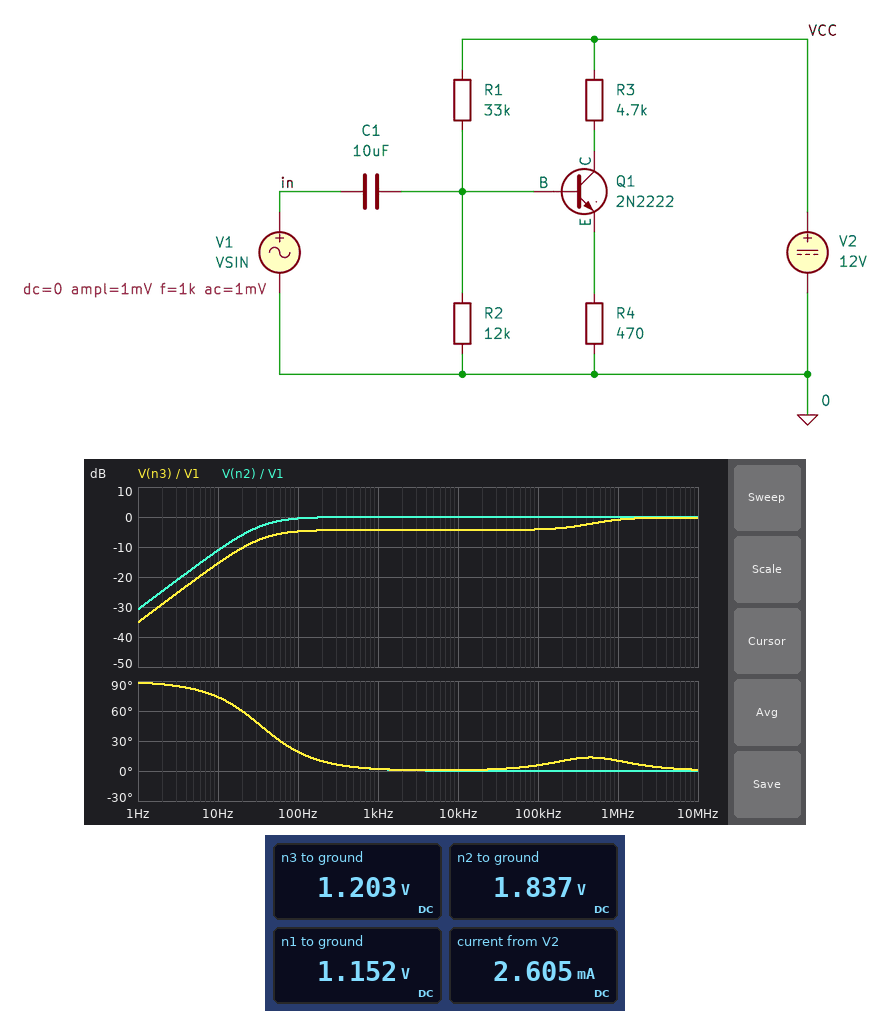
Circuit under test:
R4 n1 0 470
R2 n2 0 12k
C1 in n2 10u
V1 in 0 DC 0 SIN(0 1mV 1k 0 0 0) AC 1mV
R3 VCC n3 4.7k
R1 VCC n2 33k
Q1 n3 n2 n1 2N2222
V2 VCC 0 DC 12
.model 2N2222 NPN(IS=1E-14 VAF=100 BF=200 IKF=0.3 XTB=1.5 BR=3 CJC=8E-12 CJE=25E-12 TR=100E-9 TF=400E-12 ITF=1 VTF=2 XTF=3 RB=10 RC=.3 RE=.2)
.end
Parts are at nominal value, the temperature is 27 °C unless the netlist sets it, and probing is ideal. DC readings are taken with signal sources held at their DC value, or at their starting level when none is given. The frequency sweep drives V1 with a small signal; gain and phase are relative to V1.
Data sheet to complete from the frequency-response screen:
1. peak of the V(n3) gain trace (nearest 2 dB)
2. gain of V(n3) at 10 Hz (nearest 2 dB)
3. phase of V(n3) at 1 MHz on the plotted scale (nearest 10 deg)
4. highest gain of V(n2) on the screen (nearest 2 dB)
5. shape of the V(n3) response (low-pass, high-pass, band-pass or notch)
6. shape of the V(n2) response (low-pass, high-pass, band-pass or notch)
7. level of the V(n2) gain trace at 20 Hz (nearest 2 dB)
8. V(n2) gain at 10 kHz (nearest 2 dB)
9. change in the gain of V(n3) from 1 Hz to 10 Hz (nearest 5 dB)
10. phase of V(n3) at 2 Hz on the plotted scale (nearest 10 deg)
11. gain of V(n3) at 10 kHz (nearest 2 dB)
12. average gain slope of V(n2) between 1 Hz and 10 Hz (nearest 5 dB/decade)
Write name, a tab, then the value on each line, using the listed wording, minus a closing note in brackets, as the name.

peak of the V(n3) gain trace	0 dB
gain of V(n3) at 10 Hz	-16 dB
phase of V(n3) at 1 MHz on the plotted scale	10 deg
highest gain of V(n2) on the screen	0 dB
shape of the V(n3) response	high-pass
shape of the V(n2) response	high-pass
level of the V(n2) gain trace at 20 Hz	-6 dB
V(n2) gain at 10 kHz	0 dB
change in the gain of V(n3) from 1 Hz to 10 Hz	20 dB
phase of V(n3) at 2 Hz on the plotted scale	90 deg
gain of V(n3) at 10 kHz	-4 dB
average gain slope of V(n2) between 1 Hz and 10 Hz	20 dB/decade
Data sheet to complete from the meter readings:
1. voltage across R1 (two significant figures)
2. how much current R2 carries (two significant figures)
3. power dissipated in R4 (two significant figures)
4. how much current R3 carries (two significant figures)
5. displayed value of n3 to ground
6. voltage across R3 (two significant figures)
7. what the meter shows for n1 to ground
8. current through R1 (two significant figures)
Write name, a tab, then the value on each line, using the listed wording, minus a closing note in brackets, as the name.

voltage across R1	10 V
how much current R2 carries	150 µA
power dissipated in R4	2.8 mW
how much current R3 carries	2.3 mA
displayed value of n3 to ground	1.203 V
voltage across R3	11 V
what the meter shows for n1 to ground	1.152 V
current through R1	310 µA
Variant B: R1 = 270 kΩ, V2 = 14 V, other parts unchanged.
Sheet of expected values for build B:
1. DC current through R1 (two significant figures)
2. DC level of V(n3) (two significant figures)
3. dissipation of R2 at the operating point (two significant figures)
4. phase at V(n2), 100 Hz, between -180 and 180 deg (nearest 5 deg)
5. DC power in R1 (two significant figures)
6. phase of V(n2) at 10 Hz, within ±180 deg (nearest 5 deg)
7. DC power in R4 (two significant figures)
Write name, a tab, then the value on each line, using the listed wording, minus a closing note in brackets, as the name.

DC current through R1	50 µA
DC level of V(n3)	14 V
dissipation of R2 at the operating point	29 µW
phase at V(n2), 100 Hz, between -180 and 180 deg	0 deg
DC power in R1	670 µW
phase of V(n2) at 10 Hz, within ±180 deg	10 deg
DC power in R4	980 nW
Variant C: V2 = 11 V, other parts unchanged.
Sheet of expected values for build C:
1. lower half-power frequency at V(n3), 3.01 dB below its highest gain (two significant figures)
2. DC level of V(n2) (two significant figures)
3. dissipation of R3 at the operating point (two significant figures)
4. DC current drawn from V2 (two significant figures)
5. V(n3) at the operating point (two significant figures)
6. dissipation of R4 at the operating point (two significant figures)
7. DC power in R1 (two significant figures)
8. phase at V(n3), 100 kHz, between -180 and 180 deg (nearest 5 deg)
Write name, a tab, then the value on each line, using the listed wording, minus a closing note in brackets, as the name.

lower half-power frequency at V(n3), 3.01 dB below its highest gain	340 kHz
DC level of V(n2)	1.7 V
dissipation of R3 at the operating point	21 mW
DC current drawn from V2	2.4 mA
V(n3) at the operating point	1.1 V
dissipation of R4 at the operating point	2.4 mW
DC power in R1	2.6 mW
phase at V(n3), 100 kHz, between -180 and 180 deg	5 deg
